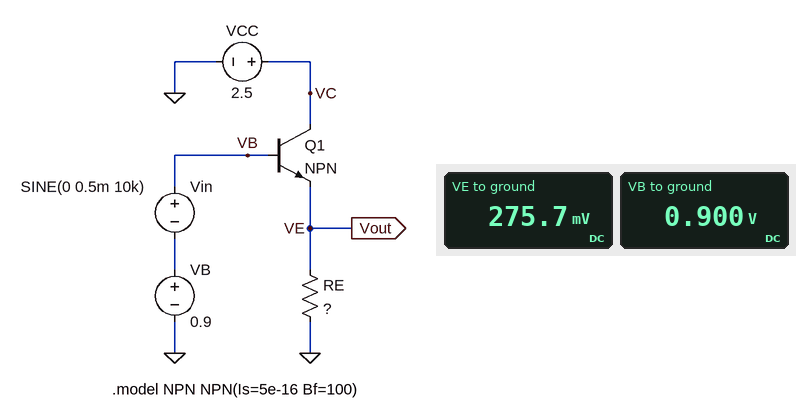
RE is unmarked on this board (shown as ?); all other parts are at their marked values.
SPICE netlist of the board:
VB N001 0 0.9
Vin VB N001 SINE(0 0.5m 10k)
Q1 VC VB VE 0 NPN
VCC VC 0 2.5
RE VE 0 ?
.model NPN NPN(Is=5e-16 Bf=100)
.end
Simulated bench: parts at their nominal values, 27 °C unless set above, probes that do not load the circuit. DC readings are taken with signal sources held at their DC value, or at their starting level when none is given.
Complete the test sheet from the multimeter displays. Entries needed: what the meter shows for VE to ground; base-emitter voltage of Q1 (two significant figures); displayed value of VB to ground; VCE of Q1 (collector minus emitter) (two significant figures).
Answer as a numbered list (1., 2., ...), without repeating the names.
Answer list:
1. 275.7 mV
2. 620 mV
3. 0.900 V
4. 2.2 V
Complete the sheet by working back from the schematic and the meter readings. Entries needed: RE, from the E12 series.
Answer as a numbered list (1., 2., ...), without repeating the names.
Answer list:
1. 18 kΩ
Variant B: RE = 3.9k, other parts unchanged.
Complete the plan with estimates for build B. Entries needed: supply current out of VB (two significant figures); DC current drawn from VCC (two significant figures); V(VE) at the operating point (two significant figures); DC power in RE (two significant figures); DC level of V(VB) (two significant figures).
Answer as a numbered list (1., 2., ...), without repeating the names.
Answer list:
1. 610 nA
2. 61 µA
3. 240 mV
4. 15 µW
5. 900 mV
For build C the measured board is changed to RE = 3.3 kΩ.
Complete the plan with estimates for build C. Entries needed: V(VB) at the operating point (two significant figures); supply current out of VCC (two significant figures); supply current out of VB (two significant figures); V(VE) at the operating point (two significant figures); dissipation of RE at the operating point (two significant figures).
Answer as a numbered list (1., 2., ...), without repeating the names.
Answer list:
1. 900 mV
2. 71 µA
3. 710 nA
4. 240 mV
5. 17 µW
